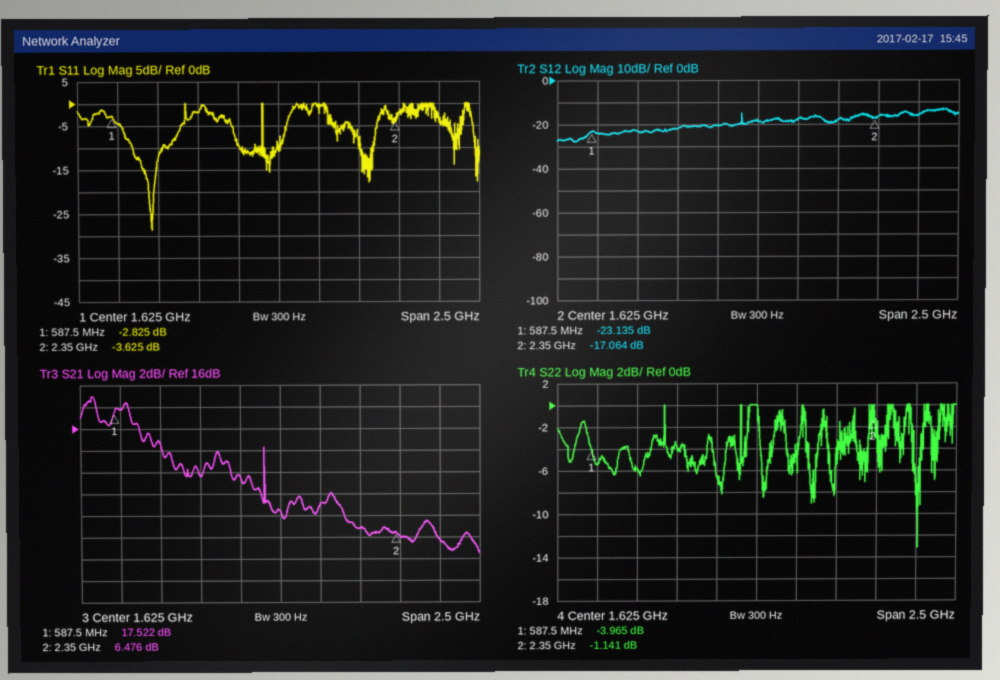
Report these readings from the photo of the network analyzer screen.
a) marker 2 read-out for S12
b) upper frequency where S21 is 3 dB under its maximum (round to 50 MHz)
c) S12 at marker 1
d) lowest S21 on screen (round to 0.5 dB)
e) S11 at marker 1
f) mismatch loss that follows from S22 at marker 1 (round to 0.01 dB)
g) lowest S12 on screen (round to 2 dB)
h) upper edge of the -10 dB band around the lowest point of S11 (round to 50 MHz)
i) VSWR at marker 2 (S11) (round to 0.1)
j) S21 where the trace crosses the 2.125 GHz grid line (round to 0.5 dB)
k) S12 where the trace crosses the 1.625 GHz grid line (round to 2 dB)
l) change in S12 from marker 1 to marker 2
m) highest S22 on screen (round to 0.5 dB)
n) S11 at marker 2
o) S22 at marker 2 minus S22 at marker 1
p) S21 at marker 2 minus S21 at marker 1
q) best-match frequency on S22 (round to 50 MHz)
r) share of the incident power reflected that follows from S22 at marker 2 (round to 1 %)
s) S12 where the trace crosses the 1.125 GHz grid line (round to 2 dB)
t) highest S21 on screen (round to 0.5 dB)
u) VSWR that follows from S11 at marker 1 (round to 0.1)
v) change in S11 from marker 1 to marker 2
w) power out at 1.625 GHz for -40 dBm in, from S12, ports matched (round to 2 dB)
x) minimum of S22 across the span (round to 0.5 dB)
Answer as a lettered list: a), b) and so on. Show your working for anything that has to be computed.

a) -17.064 dB
b) 750 MHz
c) -23.135 dB
d) 4.5 dB
e) -2.825 dB
f) −10 log10(1 − 10^(-3.965/10)) ≈ 2.23 dB
g) -28 dB
h) 900 MHz
i) (1 + 0.6588)/(1 − 0.6588) ≈ 4.9
j) 7.0 dB
k) -18 dB
l) -17.064 − (-23.135) = 6.071 dB
m) 0.0 dB
n) -3.625 dB
o) -1.141 − (-3.965) = 2.824 dB
p) 6.476 − (17.522) = -11.046 dB
q) 2.65 GHz
r) 10^(-1.141/10) ≈ 77 %
s) -22 dB
t) 19.0 dB
u) (1 + 0.7224)/(1 − 0.7224) ≈ 6.2
v) -3.625 − (-2.825) = -0.800 dB
w) -40 dBm + (-18 dB) = -58 dBm
x) -13.0 dB
